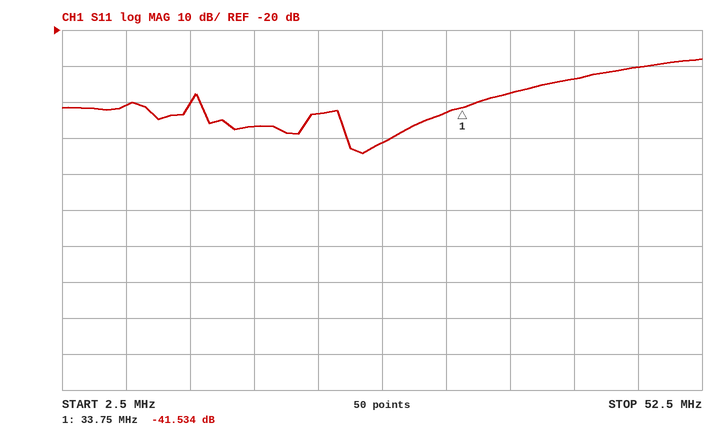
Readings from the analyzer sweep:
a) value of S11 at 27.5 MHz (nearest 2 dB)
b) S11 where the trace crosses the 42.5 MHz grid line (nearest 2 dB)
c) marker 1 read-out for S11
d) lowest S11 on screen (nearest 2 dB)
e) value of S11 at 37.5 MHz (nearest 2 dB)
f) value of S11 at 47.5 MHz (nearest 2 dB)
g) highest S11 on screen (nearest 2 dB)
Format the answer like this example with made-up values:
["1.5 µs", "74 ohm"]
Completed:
["-52 dB", "-34 dB", "-41.534 dB", "-54 dB", "-38 dB", "-30 dB", "-28 dB"]
